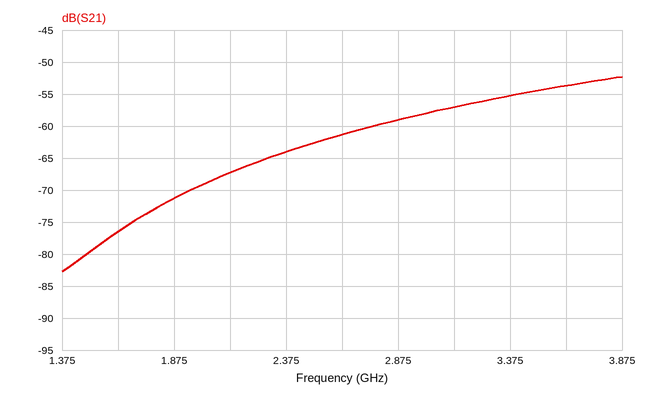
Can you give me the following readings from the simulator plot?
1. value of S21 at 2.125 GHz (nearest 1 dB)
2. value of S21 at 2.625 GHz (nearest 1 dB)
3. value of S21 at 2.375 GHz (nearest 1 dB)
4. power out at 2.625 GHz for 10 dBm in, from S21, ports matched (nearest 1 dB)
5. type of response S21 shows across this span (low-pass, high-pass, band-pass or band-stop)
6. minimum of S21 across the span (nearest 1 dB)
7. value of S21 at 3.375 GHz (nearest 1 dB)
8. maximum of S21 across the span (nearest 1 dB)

-67 dB
-61 dB
-64 dB
-51 dBm
high-pass
-83 dB
-55 dB
-52 dB
